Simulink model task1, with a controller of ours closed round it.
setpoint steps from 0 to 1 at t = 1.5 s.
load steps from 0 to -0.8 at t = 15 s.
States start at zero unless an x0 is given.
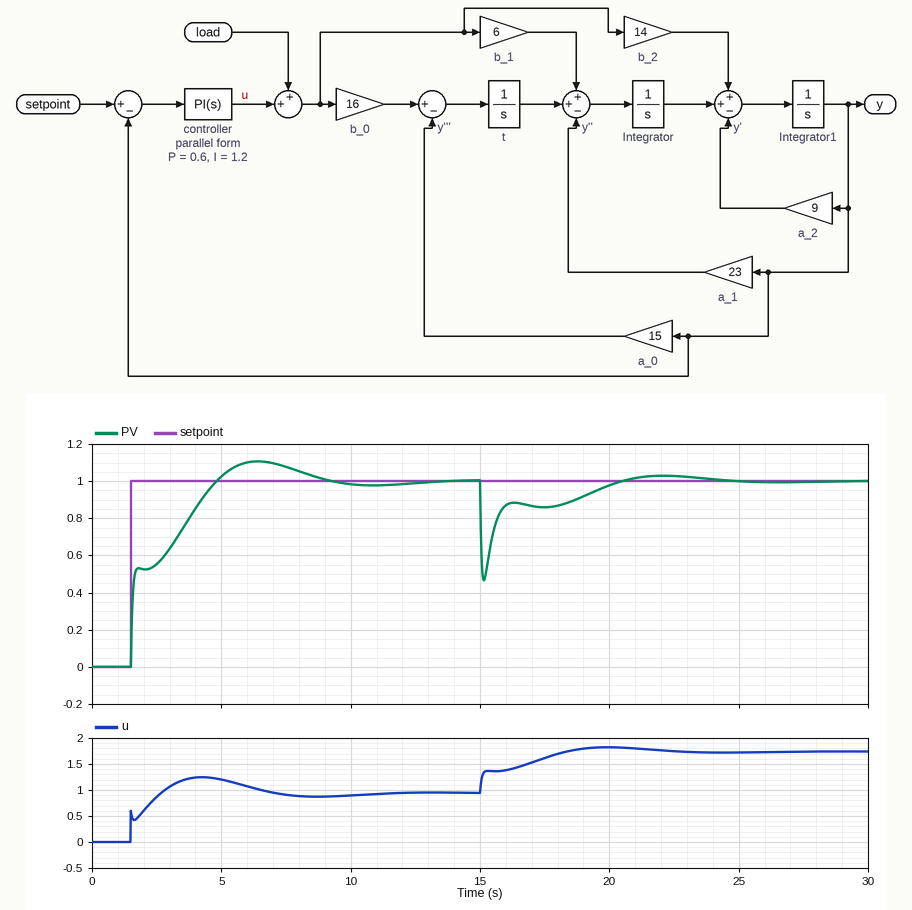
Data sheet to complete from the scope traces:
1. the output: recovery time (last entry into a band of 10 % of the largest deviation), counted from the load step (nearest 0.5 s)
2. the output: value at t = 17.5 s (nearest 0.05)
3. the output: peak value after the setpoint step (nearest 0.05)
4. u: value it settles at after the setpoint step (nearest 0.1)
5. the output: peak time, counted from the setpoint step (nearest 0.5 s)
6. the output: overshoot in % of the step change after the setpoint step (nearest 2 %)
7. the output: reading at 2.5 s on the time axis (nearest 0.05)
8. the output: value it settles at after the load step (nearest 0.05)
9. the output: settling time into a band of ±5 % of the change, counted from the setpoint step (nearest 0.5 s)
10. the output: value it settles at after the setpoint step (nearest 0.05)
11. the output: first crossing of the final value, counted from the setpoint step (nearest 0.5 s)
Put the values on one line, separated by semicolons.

4.5 s; 0.85; 1.10; 0.9; 5.0 s; 10 %; 0.55; 1.00; 6.5 s; 1.00; 3.5 s
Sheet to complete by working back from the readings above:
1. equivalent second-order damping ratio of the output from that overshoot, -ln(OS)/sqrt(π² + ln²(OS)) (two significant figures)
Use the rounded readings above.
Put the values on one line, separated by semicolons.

0.59
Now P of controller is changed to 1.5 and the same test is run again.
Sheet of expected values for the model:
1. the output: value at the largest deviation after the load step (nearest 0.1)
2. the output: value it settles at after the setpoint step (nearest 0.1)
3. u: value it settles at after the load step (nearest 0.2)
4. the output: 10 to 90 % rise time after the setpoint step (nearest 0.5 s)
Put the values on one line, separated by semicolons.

0.7; 1.0; 1.8; 3.0 s
